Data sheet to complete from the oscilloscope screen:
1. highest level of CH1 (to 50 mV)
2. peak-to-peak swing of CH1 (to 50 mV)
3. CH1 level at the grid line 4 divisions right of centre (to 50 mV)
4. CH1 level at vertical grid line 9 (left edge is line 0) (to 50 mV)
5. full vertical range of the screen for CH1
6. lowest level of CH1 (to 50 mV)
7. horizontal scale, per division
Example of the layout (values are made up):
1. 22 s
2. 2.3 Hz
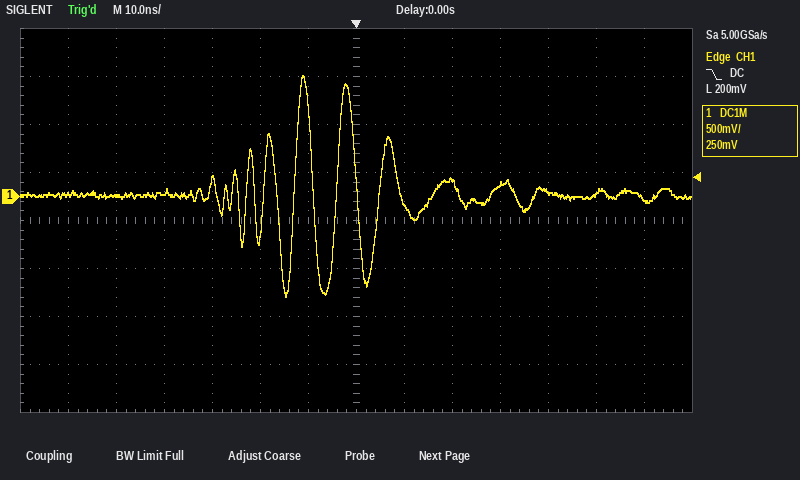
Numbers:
1. 1.25 V
2. 2.30 V
3. 50 mV
4. 200 mV
5. 4 V
6. -1.05 V
7. 10 ns
